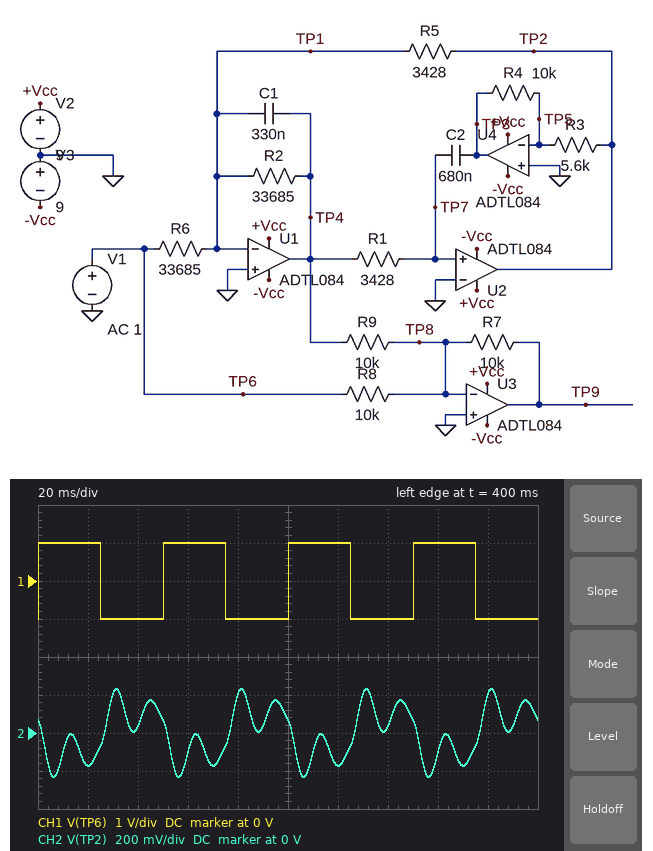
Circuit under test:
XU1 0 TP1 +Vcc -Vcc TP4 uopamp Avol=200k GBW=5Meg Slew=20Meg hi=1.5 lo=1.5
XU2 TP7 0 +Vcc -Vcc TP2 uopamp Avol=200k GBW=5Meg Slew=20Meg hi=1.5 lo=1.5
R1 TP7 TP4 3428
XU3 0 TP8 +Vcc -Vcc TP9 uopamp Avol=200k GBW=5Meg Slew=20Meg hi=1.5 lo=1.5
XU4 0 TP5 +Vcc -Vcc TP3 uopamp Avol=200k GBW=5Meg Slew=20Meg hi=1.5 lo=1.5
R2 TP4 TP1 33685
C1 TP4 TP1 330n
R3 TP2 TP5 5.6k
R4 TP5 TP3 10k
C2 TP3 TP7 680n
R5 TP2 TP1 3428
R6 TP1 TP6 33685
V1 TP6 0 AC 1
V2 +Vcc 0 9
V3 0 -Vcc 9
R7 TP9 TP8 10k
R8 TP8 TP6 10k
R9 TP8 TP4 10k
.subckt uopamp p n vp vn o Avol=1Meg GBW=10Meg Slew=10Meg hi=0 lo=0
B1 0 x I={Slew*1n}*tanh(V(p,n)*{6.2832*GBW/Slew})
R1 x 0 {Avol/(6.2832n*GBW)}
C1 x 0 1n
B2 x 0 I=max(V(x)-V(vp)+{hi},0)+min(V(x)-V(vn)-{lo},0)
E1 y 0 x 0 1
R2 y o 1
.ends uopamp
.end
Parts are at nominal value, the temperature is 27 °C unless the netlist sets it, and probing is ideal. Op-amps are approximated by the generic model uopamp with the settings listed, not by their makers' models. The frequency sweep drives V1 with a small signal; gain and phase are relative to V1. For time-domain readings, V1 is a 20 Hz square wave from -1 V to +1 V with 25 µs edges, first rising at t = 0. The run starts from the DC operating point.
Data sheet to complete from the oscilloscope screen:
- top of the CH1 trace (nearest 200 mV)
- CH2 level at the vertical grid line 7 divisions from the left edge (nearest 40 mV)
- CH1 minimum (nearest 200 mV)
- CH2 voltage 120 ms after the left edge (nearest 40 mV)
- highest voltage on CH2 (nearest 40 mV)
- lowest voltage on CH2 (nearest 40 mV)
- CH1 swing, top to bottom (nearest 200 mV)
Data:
1.0 V
40 mV
-1.0 V
-160 mV
240 mV
-240 mV
2.0 V
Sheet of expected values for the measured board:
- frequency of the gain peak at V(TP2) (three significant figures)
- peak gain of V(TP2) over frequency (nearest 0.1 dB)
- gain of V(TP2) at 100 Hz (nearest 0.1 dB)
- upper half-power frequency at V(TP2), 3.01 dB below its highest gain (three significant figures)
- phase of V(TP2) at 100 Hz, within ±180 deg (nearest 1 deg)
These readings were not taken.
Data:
72.6 Hz
-5.6 dB
-18.9 dB
79.5 Hz
17 deg
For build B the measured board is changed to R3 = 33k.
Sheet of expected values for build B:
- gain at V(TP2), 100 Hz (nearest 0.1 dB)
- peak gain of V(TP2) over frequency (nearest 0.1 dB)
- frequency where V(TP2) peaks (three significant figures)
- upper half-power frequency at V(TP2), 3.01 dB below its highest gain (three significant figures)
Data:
-16.6 dB
2.1 dB
178 Hz
185 Hz
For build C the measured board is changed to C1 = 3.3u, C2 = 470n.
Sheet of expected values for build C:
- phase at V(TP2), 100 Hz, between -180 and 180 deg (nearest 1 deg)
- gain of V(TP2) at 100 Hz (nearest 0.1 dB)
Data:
1 deg
-41.3 dB
